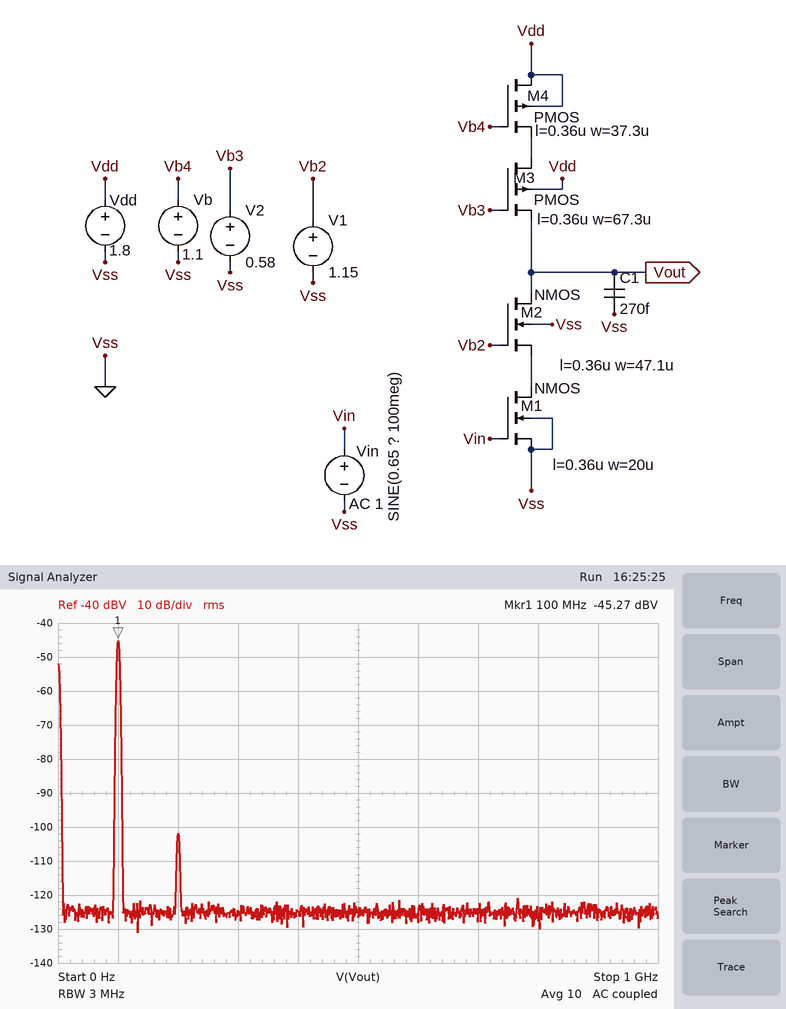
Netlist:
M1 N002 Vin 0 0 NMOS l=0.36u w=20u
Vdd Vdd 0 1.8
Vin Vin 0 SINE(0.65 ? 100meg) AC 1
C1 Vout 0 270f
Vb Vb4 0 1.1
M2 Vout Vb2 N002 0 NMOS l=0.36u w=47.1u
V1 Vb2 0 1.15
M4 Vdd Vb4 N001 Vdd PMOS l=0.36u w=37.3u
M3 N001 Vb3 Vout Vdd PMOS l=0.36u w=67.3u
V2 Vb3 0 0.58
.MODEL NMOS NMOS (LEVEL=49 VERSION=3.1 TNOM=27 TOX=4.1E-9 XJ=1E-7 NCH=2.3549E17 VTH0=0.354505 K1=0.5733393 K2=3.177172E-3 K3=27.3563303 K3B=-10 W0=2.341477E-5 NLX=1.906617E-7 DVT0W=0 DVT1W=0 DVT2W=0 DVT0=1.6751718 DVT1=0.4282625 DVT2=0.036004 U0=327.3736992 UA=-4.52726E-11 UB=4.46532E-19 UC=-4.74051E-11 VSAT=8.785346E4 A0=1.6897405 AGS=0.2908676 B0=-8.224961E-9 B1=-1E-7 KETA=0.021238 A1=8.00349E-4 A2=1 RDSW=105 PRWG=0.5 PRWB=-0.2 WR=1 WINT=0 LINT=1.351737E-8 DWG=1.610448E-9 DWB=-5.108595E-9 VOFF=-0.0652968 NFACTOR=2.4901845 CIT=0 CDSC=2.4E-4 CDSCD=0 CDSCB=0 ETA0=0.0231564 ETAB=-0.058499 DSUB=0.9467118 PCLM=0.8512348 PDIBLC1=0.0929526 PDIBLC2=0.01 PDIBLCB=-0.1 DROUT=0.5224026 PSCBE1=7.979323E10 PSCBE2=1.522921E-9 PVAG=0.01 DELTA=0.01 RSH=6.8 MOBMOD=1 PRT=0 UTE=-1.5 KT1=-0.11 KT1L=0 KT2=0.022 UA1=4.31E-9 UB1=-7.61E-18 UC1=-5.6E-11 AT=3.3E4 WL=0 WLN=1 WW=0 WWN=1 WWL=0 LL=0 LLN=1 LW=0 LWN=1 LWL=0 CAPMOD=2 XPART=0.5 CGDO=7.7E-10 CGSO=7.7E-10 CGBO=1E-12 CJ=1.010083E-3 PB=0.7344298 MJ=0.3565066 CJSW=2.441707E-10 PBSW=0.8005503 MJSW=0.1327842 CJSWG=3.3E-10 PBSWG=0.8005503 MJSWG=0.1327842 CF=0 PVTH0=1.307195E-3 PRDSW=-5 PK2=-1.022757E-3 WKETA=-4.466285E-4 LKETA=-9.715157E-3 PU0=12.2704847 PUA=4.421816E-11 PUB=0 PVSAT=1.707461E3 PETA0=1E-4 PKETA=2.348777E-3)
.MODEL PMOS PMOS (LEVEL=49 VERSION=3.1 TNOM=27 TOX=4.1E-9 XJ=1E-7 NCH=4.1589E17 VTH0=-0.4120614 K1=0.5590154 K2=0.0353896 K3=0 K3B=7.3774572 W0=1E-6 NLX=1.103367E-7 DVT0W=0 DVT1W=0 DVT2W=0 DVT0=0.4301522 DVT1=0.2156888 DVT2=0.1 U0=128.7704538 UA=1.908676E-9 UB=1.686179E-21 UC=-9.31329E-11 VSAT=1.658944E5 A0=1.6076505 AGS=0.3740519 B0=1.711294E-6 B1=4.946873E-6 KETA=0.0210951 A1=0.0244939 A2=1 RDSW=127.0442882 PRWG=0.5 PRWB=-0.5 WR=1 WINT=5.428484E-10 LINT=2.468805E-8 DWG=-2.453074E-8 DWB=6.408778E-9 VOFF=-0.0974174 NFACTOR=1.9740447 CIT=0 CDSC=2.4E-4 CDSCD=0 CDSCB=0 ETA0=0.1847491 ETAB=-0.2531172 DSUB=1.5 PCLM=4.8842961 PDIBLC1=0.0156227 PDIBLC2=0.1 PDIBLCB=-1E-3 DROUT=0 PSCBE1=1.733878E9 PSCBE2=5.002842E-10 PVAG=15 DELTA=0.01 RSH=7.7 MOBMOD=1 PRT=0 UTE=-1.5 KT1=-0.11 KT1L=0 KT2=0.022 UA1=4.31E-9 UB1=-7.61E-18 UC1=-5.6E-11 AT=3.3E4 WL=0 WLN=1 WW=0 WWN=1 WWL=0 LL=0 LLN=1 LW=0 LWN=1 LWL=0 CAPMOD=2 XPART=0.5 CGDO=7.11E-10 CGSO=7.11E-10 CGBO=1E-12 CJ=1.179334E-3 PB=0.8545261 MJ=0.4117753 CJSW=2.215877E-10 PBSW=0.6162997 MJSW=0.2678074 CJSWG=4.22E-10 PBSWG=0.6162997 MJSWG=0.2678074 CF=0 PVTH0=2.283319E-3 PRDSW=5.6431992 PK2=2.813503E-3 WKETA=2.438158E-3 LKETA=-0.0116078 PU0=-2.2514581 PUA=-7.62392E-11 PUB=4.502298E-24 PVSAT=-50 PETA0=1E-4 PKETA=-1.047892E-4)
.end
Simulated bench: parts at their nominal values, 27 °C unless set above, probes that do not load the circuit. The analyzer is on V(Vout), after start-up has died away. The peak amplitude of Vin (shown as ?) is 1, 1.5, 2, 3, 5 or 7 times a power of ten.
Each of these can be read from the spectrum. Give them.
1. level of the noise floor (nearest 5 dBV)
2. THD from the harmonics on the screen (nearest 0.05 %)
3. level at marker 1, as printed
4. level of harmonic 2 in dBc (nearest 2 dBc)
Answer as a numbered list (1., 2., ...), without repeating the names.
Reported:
1. -125 dBV
2. 0.15 %
3. -45.27 dBV
4. -56 dBc
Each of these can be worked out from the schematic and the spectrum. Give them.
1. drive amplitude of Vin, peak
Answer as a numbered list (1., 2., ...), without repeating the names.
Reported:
1. 1.5 mV
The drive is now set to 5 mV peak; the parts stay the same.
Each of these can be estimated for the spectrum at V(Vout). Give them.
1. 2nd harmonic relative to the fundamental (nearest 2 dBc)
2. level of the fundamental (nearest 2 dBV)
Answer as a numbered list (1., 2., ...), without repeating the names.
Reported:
1. -46 dBc
2. -34 dBV
